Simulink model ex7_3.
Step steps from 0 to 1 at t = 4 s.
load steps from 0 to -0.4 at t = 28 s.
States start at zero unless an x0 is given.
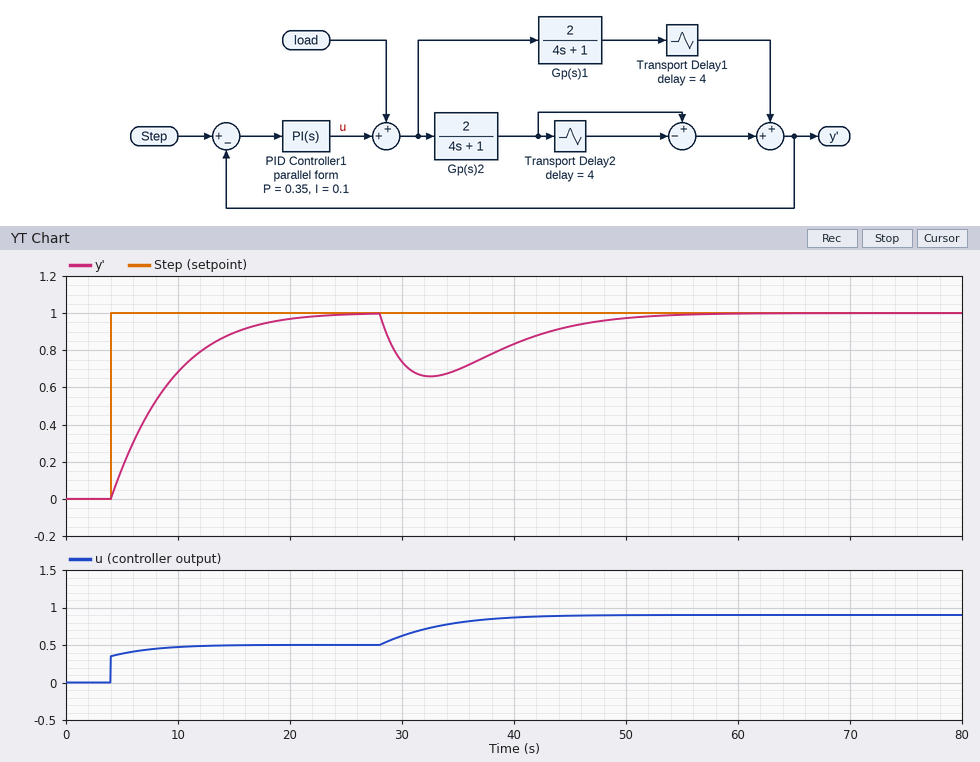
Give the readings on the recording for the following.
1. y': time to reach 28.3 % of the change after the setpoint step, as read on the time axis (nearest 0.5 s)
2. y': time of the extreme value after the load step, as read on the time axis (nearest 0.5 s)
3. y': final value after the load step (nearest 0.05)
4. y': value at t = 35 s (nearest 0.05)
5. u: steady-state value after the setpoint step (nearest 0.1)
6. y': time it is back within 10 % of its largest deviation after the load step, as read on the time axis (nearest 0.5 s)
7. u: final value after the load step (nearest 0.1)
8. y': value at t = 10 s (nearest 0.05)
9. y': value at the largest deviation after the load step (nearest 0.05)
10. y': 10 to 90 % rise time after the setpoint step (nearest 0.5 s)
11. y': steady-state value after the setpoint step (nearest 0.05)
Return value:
6.0 s
32.5 s
1.00
0.70
0.5
49.0 s
0.9
0.70
0.65
10.5 s
1.00
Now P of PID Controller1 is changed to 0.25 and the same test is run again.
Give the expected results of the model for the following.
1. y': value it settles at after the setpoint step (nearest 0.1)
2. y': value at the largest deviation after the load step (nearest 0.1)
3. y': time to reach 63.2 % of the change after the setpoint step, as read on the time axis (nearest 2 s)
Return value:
1.0
0.6
10 s
